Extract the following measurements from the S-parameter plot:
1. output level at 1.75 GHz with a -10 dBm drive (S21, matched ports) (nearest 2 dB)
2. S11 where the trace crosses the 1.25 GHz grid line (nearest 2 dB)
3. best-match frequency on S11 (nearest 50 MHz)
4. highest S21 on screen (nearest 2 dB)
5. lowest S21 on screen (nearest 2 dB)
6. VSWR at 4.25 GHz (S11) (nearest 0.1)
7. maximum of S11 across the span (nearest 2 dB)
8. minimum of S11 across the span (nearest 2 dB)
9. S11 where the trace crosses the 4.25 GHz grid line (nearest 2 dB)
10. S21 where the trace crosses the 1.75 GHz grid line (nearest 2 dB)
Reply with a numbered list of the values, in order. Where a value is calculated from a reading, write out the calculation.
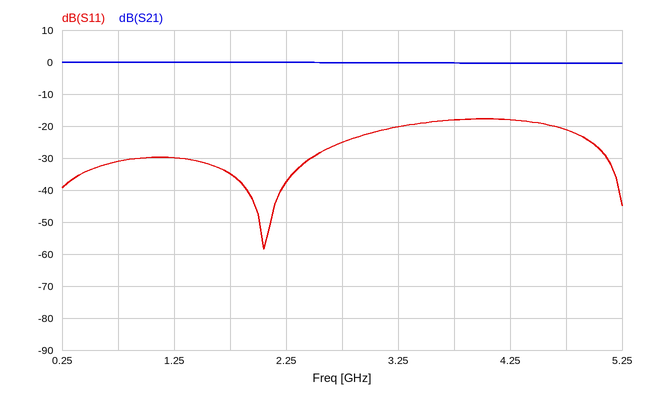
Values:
1. -10 dBm + (0 dB) = -10 dBm
2. -30 dB
3. 2.05 GHz
4. 0 dB
5. 0 dB
6. |Γ| = 10^(-18/20) = 0.1259; VSWR = (1 + 0.1259)/(1 − 0.1259) ≈ 1.3
7. -18 dB
8. -58 dB
9. -18 dB
10. 0 dB
